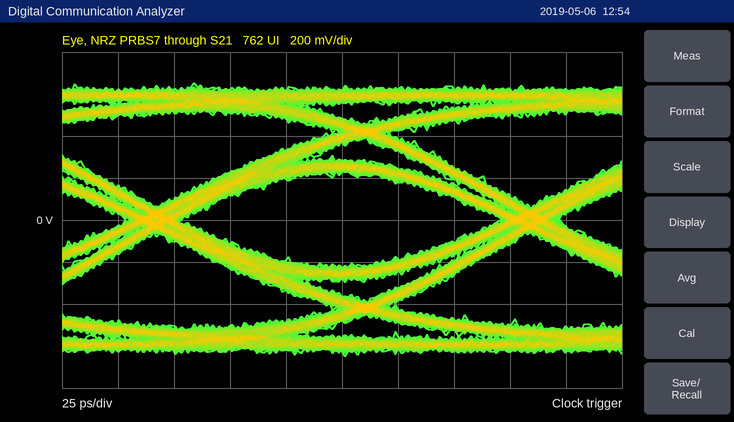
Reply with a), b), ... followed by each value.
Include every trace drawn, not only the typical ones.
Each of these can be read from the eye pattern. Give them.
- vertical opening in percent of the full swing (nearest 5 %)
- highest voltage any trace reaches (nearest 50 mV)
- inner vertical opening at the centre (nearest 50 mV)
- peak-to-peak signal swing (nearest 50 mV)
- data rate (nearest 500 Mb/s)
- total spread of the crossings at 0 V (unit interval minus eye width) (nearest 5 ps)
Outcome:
a) 35 %
b) 650 mV
c) 450 mV
d) 1.30 V
e) 6.0 Gb/s
f) 25 ps
